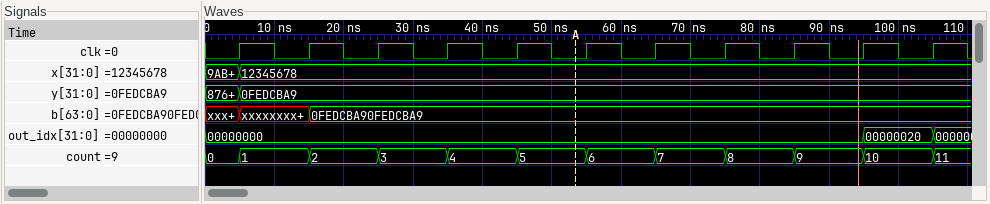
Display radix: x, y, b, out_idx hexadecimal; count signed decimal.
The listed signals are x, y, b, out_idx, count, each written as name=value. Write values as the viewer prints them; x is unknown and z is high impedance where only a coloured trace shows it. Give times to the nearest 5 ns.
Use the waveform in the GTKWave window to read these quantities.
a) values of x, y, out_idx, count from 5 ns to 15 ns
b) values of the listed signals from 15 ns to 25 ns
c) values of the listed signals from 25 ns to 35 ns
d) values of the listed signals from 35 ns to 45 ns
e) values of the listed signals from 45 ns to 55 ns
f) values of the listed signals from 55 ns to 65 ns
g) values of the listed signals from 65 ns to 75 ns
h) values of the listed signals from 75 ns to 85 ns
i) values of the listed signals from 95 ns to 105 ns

x=12345678, y=0FEDCBA9, out_idx=00000000, count=1
x=12345678, y=0FEDCBA9, b=0FEDCBA90FEDCBA9, out_idx=00000000, count=2
x=12345678, y=0FEDCBA9, b=0FEDCBA90FEDCBA9, out_idx=00000000, count=3
x=12345678, y=0FEDCBA9, b=0FEDCBA90FEDCBA9, out_idx=00000000, count=4
x=12345678, y=0FEDCBA9, b=0FEDCBA90FEDCBA9, out_idx=00000000, count=5
x=12345678, y=0FEDCBA9, b=0FEDCBA90FEDCBA9, out_idx=00000000, count=6
x=12345678, y=0FEDCBA9, b=0FEDCBA90FEDCBA9, out_idx=00000000, count=7
x=12345678, y=0FEDCBA9, b=0FEDCBA90FEDCBA9, out_idx=00000000, count=8
x=12345678, y=0FEDCBA9, b=0FEDCBA90FEDCBA9, out_idx=00000020, count=10
